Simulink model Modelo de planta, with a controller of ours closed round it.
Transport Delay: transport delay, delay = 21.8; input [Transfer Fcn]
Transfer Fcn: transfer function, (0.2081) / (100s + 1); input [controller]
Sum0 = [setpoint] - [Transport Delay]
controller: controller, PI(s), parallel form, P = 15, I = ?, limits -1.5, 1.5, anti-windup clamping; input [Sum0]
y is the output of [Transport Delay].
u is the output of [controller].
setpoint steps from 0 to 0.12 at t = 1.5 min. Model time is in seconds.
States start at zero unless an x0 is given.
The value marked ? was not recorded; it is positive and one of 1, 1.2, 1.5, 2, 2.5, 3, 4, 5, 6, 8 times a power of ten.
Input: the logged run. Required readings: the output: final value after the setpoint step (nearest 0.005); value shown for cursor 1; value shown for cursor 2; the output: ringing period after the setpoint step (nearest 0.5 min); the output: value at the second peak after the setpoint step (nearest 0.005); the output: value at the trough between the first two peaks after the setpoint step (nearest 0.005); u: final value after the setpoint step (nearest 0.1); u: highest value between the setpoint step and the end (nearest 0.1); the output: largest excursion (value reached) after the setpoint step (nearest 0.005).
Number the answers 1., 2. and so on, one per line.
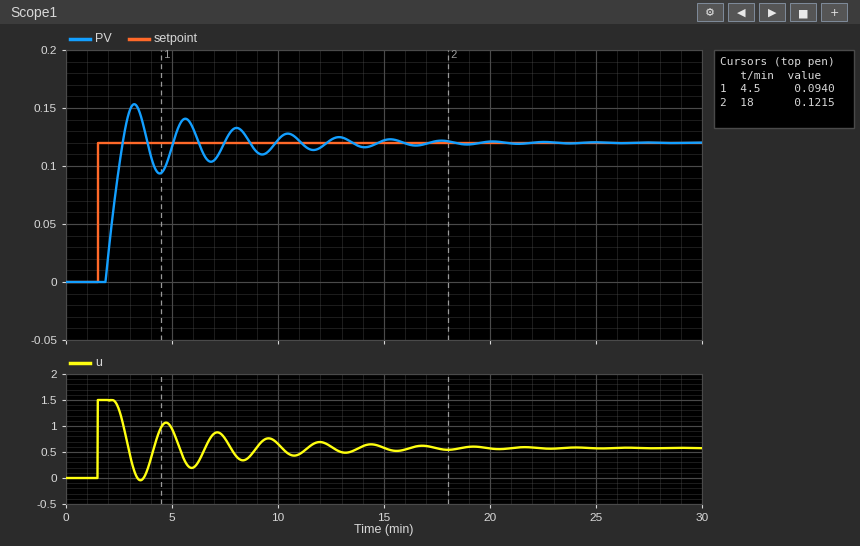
1. 0.120
2. 0.0940
3. 0.1215
4. 2.5 min
5. 0.140
6. 0.095
7. 0.6
8. 1.5
9. 0.155
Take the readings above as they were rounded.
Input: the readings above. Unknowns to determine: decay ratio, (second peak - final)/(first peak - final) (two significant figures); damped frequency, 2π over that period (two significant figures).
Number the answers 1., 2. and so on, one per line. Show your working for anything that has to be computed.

1. (0.14 - 0.12) / (0.155 - 0.12) = 0.57
2. 2π / 2.5 = 2.5 rad/min
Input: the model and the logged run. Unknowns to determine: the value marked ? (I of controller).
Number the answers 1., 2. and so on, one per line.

1. 0.6
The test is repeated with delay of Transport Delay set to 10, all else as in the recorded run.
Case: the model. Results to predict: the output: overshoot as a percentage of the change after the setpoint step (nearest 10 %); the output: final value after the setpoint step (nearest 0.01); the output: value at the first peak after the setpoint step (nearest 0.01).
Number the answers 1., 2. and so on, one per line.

1. 20 %
2. 0.12
3. 0.14
